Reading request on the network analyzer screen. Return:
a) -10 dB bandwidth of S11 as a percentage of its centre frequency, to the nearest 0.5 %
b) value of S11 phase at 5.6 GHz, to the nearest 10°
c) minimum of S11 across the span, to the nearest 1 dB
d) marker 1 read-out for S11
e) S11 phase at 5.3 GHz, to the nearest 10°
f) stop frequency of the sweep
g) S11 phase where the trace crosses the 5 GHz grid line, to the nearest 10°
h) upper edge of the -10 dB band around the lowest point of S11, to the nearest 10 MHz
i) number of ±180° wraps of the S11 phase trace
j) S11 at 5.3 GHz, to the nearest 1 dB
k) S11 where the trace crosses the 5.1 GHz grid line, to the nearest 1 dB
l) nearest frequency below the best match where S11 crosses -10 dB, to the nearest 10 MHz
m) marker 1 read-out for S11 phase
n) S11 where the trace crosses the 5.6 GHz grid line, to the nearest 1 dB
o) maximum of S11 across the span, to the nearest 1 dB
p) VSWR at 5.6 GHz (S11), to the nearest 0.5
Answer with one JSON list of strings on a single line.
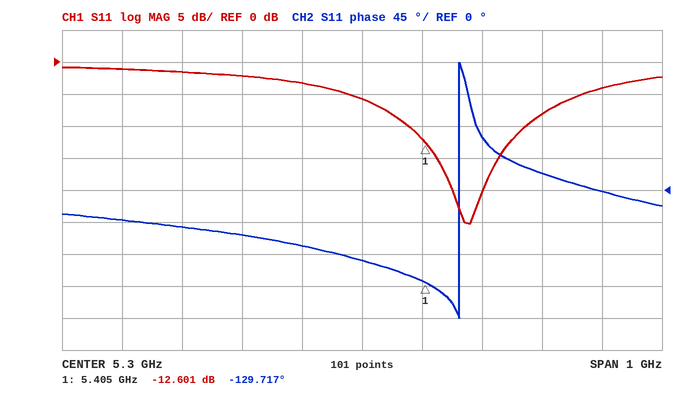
["3.5 %", "20°", "-25 dB", "-12.601 dB", "-100°", "5.8 GHz", "-50°", "5.57 GHz", "1", "-6 dB", "-2 dB", "5.38 GHz", "-129.717°", "-8 dB", "-1 dB", "2.5"]
